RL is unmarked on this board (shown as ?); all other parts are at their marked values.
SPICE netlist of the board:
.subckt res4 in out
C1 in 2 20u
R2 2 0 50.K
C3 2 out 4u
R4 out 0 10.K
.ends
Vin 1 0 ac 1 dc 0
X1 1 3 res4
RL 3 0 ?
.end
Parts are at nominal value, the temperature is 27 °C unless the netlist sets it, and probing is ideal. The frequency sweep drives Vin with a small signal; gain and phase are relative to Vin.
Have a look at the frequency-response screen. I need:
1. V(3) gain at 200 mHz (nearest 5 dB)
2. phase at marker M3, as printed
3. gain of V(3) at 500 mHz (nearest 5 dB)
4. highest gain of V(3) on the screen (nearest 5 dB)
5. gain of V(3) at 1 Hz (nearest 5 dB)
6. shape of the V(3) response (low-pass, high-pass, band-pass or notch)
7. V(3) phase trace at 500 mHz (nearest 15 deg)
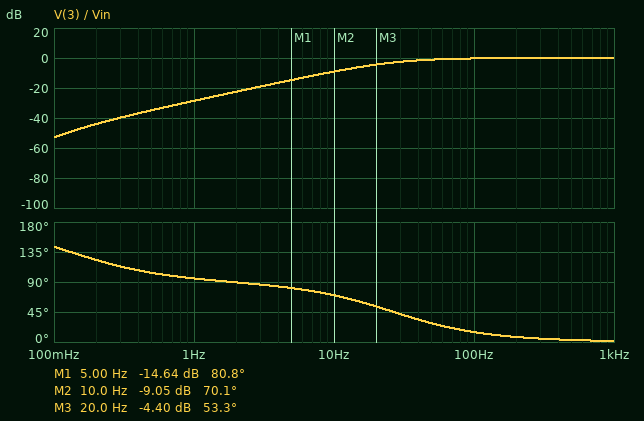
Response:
-45 dB
53.3 deg
-35 dB
0 dB
-30 dB
high-pass
105 deg
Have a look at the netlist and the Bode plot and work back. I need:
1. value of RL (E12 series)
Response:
2.2 kΩ
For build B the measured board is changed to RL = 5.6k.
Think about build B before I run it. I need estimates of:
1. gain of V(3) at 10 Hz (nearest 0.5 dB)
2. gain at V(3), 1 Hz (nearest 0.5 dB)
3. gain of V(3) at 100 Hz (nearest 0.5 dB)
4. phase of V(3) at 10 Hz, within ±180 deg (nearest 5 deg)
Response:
-4.5 dB
-22.5 dB
0 dB
55 deg
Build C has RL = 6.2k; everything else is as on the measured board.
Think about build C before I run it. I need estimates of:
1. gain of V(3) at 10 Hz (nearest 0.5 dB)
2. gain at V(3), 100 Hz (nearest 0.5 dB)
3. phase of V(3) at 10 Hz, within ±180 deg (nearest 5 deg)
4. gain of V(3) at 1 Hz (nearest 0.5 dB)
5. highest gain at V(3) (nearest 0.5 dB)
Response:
-4.0 dB
0 dB
50 deg
-22.0 dB
0 dB
